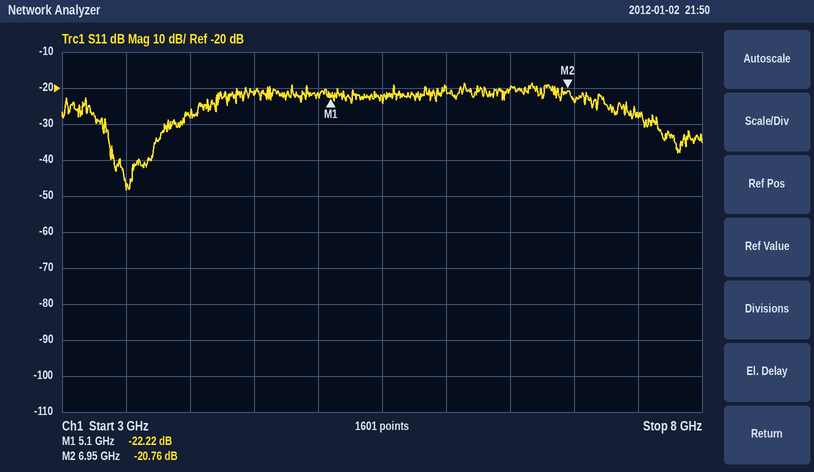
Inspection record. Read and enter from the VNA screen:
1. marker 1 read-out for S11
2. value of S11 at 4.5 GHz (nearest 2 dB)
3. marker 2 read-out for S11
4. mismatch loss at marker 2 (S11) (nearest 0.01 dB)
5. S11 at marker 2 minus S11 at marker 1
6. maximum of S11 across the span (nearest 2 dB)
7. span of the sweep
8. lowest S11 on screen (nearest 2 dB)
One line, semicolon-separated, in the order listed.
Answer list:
-22.22 dB; -22 dB; -20.76 dB; 0.04 dB; 1.46 dB; -18 dB; 5 GHz; -48 dB
